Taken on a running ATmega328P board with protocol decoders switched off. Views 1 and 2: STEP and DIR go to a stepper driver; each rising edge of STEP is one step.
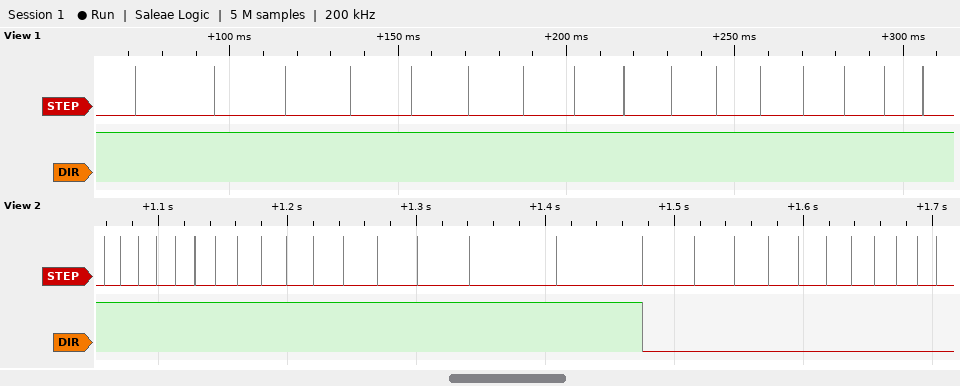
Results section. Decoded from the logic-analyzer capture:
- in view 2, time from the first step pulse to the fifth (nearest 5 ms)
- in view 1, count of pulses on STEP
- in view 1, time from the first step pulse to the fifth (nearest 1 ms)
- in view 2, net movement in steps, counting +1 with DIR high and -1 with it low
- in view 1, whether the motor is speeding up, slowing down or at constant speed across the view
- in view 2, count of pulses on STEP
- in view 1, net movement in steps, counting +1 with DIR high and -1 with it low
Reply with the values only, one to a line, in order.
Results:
55 ms
16
82 ms
+5
speeding up
27
+16
